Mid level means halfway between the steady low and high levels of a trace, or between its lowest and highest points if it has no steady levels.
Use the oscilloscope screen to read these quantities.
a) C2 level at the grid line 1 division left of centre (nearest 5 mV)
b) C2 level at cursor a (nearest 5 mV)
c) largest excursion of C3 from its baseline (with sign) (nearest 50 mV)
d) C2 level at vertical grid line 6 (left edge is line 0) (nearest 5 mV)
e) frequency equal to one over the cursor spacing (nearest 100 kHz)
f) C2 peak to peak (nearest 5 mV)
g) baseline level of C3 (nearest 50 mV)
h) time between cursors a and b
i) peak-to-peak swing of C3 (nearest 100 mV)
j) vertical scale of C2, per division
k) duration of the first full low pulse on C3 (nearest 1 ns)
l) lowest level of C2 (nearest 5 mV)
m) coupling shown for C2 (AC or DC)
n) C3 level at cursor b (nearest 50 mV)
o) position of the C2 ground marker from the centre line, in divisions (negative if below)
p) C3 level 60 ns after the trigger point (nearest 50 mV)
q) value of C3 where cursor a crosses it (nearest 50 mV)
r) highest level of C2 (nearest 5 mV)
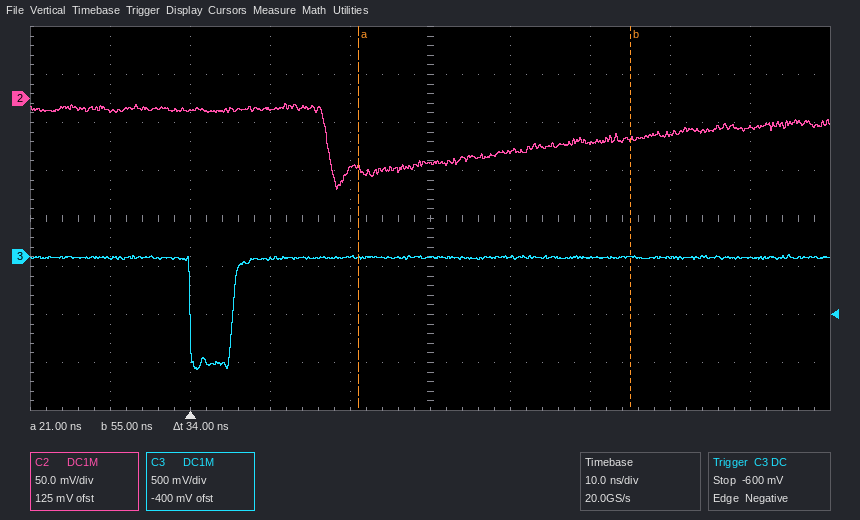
-75 mV
-75 mV
-1.15 V
-55 mV
29.4 MHz
90 mV
0 mV
34 ns
1.20 V
50 mV
5 ns
-95 mV
DC
0 mV
+2.5 div
0 mV
0 mV
-5 mV
